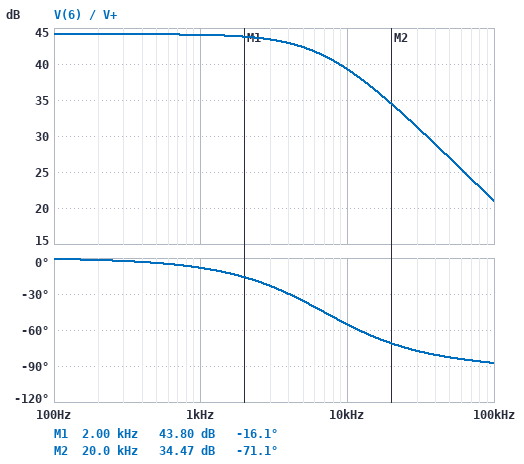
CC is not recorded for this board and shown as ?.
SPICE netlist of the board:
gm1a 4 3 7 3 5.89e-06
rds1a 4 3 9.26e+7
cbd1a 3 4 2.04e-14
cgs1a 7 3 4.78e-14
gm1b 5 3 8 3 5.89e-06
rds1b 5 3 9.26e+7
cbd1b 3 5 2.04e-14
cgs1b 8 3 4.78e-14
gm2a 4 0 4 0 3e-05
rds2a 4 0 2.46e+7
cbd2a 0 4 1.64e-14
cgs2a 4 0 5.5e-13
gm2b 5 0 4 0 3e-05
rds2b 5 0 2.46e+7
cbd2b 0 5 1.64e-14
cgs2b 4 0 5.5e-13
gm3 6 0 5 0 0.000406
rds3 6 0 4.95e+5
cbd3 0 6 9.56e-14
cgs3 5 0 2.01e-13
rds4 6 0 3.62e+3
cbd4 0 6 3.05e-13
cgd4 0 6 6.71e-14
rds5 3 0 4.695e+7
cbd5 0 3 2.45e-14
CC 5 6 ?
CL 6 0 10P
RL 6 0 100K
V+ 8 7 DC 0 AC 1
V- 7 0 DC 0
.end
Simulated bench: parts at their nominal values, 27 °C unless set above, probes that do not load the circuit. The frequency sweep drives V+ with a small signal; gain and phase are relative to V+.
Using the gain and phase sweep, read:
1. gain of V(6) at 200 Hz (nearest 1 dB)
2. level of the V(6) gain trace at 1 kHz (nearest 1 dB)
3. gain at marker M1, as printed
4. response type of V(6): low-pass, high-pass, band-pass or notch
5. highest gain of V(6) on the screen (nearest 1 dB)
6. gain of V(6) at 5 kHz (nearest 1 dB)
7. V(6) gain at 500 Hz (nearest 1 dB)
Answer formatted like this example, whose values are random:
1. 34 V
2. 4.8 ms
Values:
1. 44 dB
2. 44 dB
3. 43.80 dB
4. low-pass
5. 44 dB
6. 42 dB
7. 44 dB
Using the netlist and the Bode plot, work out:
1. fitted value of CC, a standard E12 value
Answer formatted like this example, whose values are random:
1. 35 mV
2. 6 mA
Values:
1. 390 fF
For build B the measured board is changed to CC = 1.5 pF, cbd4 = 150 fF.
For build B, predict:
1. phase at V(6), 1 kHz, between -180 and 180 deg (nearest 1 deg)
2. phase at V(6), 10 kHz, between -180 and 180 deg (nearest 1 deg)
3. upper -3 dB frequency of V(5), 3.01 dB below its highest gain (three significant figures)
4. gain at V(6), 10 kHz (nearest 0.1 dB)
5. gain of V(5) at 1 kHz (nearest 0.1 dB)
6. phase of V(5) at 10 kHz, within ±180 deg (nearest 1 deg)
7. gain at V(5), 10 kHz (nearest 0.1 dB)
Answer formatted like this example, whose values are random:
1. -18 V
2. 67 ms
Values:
1. -25 deg
2. -78 deg
3. 2.13 kHz
4. 30.5 dB
5. 40.3 dB
6. 102 deg
7. 27.5 dB
